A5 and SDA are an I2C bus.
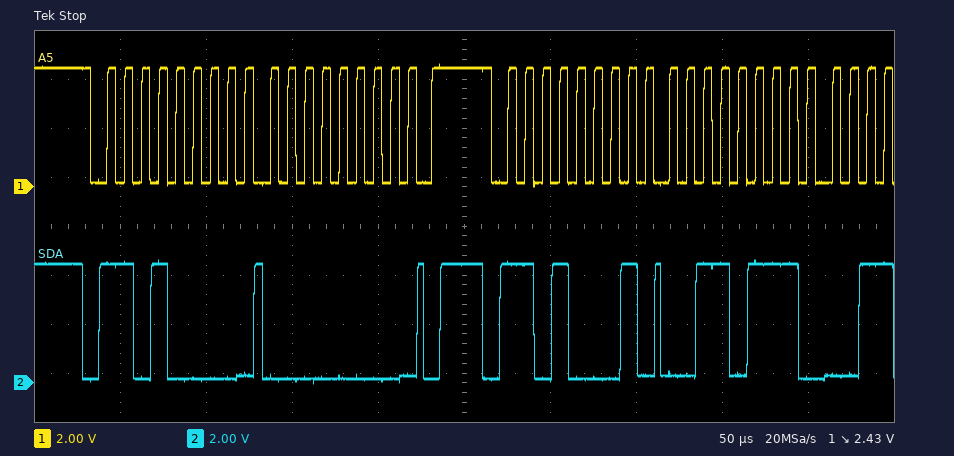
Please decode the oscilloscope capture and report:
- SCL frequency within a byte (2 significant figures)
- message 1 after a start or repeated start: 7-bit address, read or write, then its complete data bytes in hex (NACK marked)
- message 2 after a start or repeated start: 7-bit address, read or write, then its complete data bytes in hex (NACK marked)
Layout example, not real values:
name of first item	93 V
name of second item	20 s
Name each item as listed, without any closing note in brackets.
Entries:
SCL frequency within a byte	100 kHz
message 1 after a start or repeated start: 7-bit address, read or write, then its complete data bytes in hex	0x68 write: 00
message 2 after a start or repeated start: 7-bit address, read or write, then its complete data bytes in hex	0x68 read: 37
